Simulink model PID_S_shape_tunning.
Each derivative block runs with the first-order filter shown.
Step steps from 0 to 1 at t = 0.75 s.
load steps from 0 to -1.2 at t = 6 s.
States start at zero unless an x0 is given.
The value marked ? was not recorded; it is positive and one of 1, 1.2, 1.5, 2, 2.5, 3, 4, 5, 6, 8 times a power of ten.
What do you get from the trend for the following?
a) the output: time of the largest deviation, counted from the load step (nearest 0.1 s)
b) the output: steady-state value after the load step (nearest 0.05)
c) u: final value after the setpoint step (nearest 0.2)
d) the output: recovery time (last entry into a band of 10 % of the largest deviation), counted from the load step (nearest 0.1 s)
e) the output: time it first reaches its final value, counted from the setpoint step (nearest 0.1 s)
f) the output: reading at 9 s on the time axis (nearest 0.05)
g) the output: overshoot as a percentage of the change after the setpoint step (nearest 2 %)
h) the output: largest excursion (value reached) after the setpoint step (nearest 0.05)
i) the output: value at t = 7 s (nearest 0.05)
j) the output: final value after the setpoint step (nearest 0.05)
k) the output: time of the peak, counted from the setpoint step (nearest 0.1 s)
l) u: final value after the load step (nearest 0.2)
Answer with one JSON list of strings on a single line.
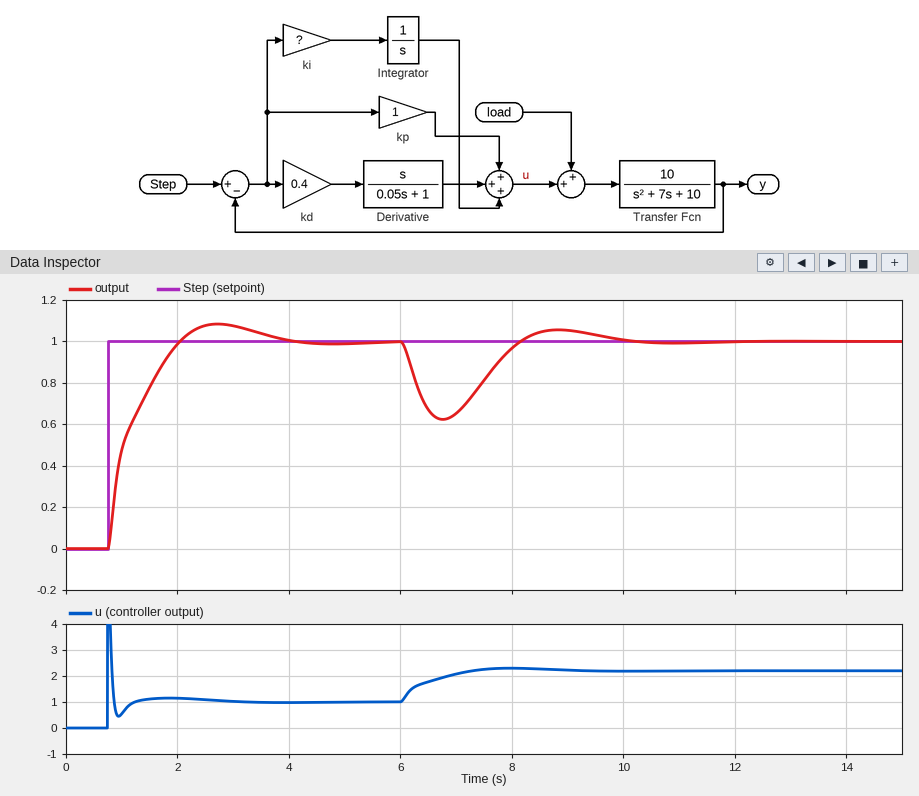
["0.8 s", "1.00", "1.0", "3.4 s", "1.3 s", "1.05", "8 %", "1.10", "0.65", "1.00", "2.0 s", "2.2"]
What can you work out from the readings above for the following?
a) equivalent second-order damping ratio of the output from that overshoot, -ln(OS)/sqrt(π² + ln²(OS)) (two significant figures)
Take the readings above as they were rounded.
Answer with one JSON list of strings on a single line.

["0.63"]
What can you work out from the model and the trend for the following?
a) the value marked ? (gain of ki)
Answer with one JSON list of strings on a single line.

["3"]
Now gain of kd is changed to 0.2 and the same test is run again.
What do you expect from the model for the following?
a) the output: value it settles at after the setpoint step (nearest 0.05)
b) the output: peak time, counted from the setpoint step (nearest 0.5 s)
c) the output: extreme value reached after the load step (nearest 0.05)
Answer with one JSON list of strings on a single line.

["1.00", "1.5 s", "0.60"]
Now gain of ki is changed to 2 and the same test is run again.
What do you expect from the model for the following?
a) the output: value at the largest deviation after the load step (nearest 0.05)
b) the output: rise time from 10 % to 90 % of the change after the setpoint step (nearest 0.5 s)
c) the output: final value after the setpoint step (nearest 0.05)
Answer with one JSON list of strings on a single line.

["0.60", "1.5 s", "1.00"]
